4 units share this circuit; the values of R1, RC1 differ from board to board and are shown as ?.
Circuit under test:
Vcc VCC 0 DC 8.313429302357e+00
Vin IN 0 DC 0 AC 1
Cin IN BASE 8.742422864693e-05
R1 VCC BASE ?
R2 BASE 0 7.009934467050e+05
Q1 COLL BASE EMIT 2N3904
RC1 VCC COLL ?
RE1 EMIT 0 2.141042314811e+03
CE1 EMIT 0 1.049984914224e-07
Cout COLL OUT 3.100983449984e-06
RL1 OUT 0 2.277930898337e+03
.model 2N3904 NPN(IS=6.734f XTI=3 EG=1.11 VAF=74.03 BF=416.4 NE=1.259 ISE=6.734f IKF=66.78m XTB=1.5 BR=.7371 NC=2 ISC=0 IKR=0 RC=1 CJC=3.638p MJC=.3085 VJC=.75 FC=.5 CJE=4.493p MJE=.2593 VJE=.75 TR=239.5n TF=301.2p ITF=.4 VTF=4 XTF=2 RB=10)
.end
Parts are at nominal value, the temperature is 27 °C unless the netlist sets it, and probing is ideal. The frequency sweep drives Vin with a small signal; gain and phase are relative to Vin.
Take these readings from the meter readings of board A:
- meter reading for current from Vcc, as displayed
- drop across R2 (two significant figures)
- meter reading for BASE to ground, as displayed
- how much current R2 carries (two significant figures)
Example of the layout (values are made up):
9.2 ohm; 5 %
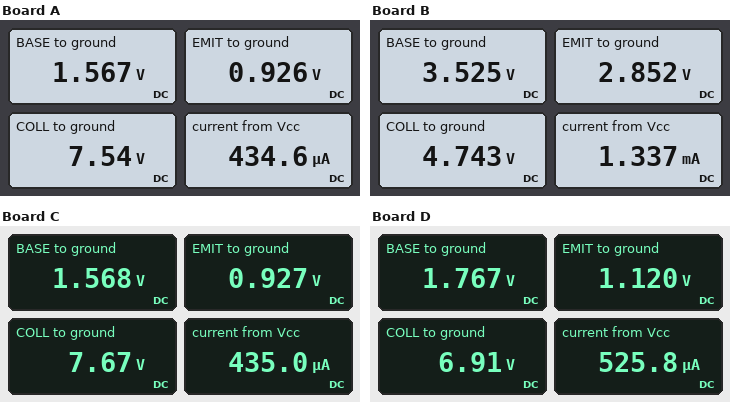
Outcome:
434.6 µA; 1.6 V; 1.567 V; 2.2 µA
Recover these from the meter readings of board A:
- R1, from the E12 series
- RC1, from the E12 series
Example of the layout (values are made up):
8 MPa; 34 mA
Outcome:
1.2 MΩ; 1.8 kΩ
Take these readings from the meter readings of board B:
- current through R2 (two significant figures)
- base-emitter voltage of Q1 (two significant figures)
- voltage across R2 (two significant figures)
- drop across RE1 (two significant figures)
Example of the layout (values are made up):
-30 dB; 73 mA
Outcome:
5.0 µA; 670 mV; 3.5 V; 2.9 V
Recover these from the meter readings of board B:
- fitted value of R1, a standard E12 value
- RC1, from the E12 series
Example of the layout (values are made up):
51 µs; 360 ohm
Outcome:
330 kΩ; 2.7 kΩ
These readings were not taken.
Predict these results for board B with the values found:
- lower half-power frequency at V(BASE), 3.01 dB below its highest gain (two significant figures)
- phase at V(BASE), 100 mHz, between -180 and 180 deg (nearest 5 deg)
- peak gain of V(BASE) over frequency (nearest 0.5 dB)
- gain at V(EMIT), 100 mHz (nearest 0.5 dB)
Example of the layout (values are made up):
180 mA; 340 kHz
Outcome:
14 mHz; 10 deg; 0 dB; 0 dB
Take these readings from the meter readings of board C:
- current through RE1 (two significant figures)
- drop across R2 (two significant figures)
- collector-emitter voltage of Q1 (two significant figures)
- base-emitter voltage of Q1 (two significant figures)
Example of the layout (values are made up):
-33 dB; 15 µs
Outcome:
430 µA; 1.6 V; 6.7 V; 640 mV
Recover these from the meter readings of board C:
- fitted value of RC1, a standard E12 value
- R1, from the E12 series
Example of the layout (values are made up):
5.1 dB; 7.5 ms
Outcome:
1.5 kΩ; 1.2 MΩ
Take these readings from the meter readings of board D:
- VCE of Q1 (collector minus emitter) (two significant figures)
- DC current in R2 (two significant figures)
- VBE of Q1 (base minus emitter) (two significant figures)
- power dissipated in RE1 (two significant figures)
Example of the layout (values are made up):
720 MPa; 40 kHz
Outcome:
5.8 V; 2.5 µA; 650 mV; 590 µW
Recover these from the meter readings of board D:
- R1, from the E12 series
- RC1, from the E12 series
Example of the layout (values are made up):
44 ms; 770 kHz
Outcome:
1 MΩ; 2.7 kΩ
